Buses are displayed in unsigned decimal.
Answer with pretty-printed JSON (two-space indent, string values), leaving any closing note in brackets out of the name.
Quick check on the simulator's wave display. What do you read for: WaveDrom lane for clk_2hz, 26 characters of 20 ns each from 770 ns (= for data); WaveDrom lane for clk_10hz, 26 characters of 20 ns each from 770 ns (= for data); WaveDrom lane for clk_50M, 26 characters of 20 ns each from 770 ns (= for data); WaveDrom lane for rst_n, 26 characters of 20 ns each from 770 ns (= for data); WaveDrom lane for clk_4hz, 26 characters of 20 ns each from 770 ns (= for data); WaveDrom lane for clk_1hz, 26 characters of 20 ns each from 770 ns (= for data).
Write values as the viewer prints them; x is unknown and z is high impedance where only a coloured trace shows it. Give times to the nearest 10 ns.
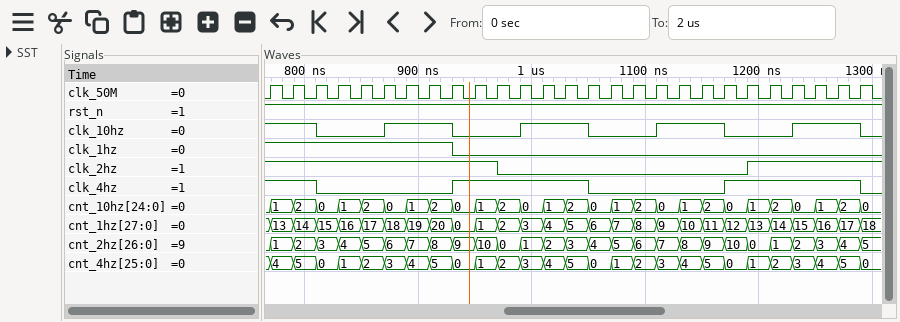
{
  "WaveDrom lane for clk_2hz, 26 characters of 20 ns each from 770 ns": "{name: 'clk_2hz', wave: '1.........0..........1....'}",
  "WaveDrom lane for clk_10hz, 26 characters of 20 ns each from 770 ns": "{name: 'clk_10hz', wave: '1.0..1..0..1..0..1..0..1..'}",
  "WaveDrom lane for clk_50M, 26 characters of 20 ns each from 770 ns": "{name: 'clk_50M', wave: 'p.........................'}",
  "WaveDrom lane for rst_n, 26 characters of 20 ns each from 770 ns": "{name: 'rst_n', wave: '1.........................'}",
  "WaveDrom lane for clk_4hz, 26 characters of 20 ns each from 770 ns": "{name: 'clk_4hz', wave: '1.0.....1.....0.....1.....'}",
  "WaveDrom lane for clk_1hz, 26 characters of 20 ns each from 770 ns": "{name: 'clk_1hz', wave: '1.......0.................'}"
}
